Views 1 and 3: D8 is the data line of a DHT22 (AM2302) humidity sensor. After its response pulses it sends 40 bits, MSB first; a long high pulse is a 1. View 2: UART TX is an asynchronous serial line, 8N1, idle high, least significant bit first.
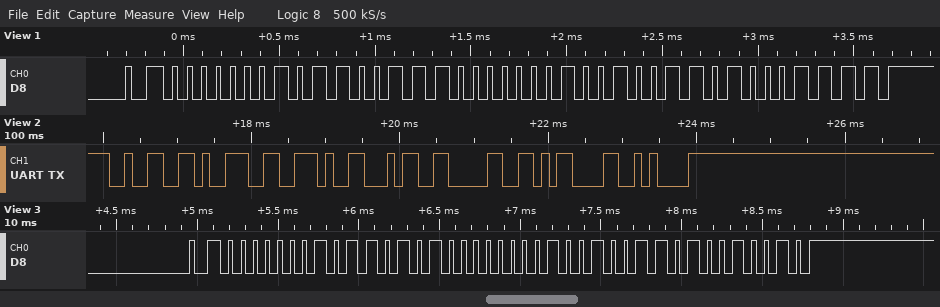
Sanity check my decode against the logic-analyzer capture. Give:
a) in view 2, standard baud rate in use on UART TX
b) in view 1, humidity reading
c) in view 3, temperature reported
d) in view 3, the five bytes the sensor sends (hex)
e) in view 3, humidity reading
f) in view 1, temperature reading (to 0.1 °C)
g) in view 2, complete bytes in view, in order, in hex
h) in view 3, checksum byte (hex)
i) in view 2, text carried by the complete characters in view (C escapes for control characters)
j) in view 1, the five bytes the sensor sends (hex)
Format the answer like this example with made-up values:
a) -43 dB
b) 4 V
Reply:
a) 9600 baud
b) 35.9 %
c) 29.4 °C
d) 01 6A 01 26 92
e) 36.2 %
f) 29.4 °C
g) 0x32 0x39 0x2E 0x34 0x30 0x0D 0x0A
h) 0x92
i) "29.40\r\n"
j) 01 67 01 26 8F
